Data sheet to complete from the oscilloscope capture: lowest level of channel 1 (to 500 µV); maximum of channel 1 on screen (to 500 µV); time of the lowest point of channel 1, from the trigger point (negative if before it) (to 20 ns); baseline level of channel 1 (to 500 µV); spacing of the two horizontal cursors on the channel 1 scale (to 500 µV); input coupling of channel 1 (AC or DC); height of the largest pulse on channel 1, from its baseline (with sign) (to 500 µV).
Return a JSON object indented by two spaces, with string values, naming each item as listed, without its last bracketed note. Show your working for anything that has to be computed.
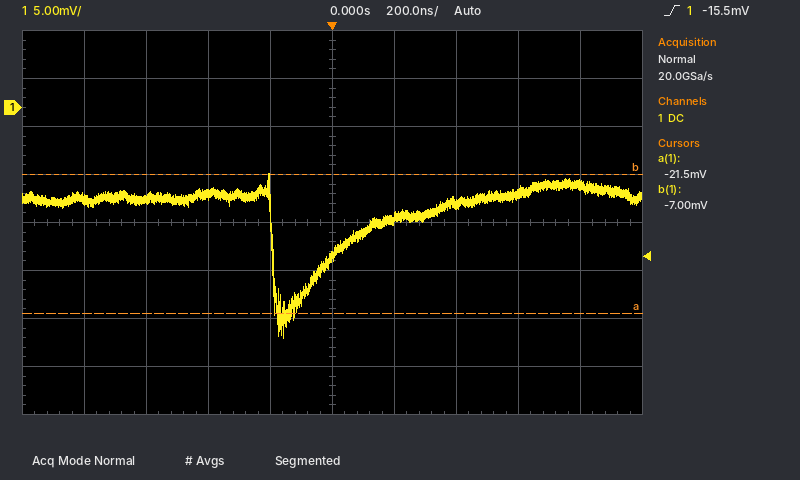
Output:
{
  "lowest level of channel 1": "-24.0 mV",
  "maximum of channel 1 on screen": "-7.0 mV",
  "time of the lowest point of channel 1, from the trigger point (negative if before it)": "-160 ns",
  "baseline level of channel 1": "-9.5 mV",
  "spacing of the two horizontal cursors on the channel 1 scale": "14.5 mV",
  "input coupling of channel 1": "DC",
  "height of the largest pulse on channel 1, from its baseline (with sign)": "-24.0 mV − (-9.5 mV) = -14.5 mV"
}
